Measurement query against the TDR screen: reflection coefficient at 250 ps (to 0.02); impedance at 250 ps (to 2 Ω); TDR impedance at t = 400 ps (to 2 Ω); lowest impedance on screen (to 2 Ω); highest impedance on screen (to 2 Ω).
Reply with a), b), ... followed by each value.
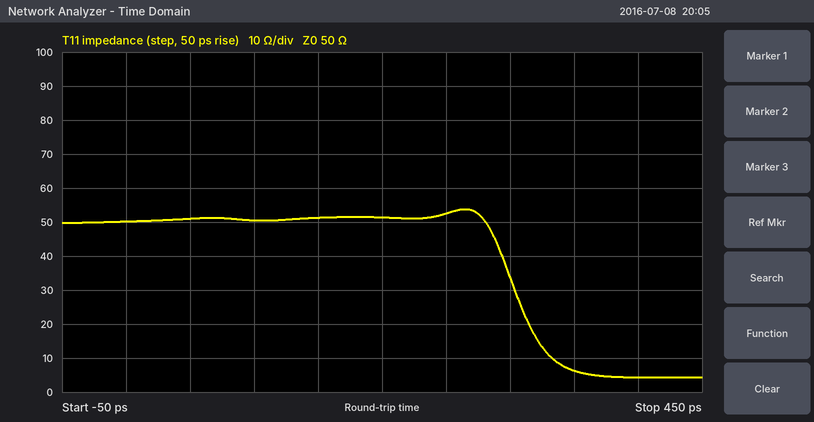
a) +0.02
b) 52 Ω
c) 4 Ω
d) 4 Ω
e) 54 Ω
